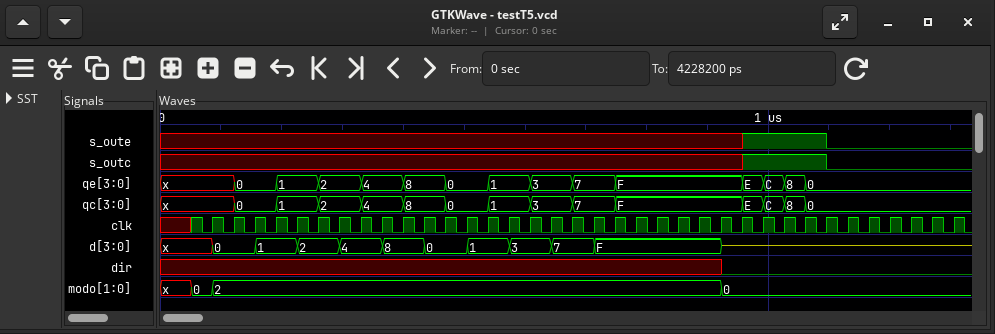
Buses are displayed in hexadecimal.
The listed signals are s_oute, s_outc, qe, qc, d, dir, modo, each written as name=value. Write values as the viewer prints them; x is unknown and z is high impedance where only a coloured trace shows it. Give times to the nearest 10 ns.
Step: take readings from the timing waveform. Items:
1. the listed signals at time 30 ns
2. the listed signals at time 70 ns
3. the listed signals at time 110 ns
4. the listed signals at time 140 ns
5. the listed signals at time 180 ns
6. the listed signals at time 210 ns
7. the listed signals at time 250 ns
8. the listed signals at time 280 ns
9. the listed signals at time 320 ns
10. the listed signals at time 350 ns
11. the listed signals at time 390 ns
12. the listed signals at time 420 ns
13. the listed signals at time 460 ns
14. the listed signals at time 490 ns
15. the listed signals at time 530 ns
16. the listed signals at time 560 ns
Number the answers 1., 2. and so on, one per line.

1. s_oute=x, s_outc=x, qe=x, qc=x, d=x, dir=x, modo=x
2. s_oute=x, s_outc=x, qe=x, qc=x, d=x, dir=x, modo=0
3. s_oute=x, s_outc=x, qe=x, qc=x, d=0, dir=x, modo=2
4. s_oute=x, s_outc=x, qe=0, qc=0, d=0, dir=x, modo=2
5. s_oute=x, s_outc=x, qe=0, qc=0, d=1, dir=x, modo=2
6. s_oute=x, s_outc=x, qe=1, qc=1, d=1, dir=x, modo=2
7. s_oute=x, s_outc=x, qe=1, qc=1, d=2, dir=x, modo=2
8. s_oute=x, s_outc=x, qe=2, qc=2, d=2, dir=x, modo=2
9. s_oute=x, s_outc=x, qe=2, qc=2, d=4, dir=x, modo=2
10. s_oute=x, s_outc=x, qe=4, qc=4, d=4, dir=x, modo=2
11. s_oute=x, s_outc=x, qe=4, qc=4, d=8, dir=x, modo=2
12. s_oute=x, s_outc=x, qe=8, qc=8, d=8, dir=x, modo=2
13. s_oute=x, s_outc=x, qe=8, qc=8, d=0, dir=x, modo=2
14. s_oute=x, s_outc=x, qe=0, qc=0, d=0, dir=x, modo=2
15. s_oute=x, s_outc=x, qe=0, qc=0, d=1, dir=x, modo=2
16. s_oute=x, s_outc=x, qe=1, qc=1, d=1, dir=x, modo=2
